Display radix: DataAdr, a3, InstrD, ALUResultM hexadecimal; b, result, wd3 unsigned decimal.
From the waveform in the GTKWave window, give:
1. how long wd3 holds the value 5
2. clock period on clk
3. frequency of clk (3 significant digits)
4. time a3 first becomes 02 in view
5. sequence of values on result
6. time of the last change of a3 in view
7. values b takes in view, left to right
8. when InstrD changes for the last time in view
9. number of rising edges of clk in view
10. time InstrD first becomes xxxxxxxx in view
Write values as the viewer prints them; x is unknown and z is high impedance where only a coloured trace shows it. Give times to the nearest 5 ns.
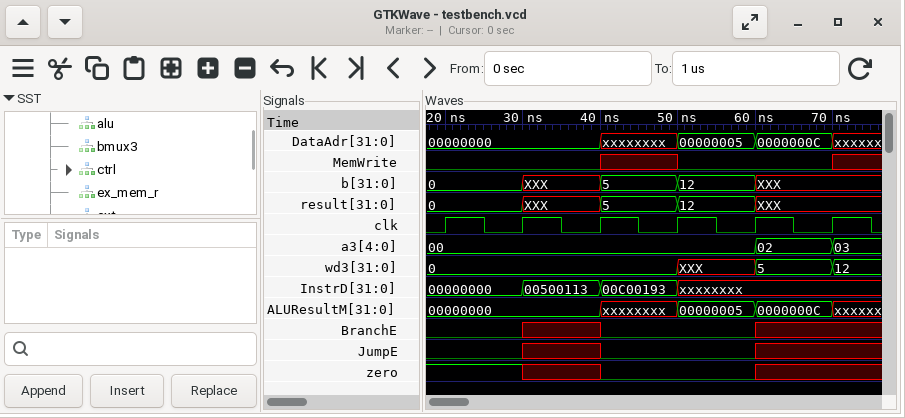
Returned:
10 ns
10 ns
100 MHz
60 ns
0, XXX, 5, 12, XXX
70 ns
0, XXX, 5, 12, XXX
50 ns
6
50 ns
